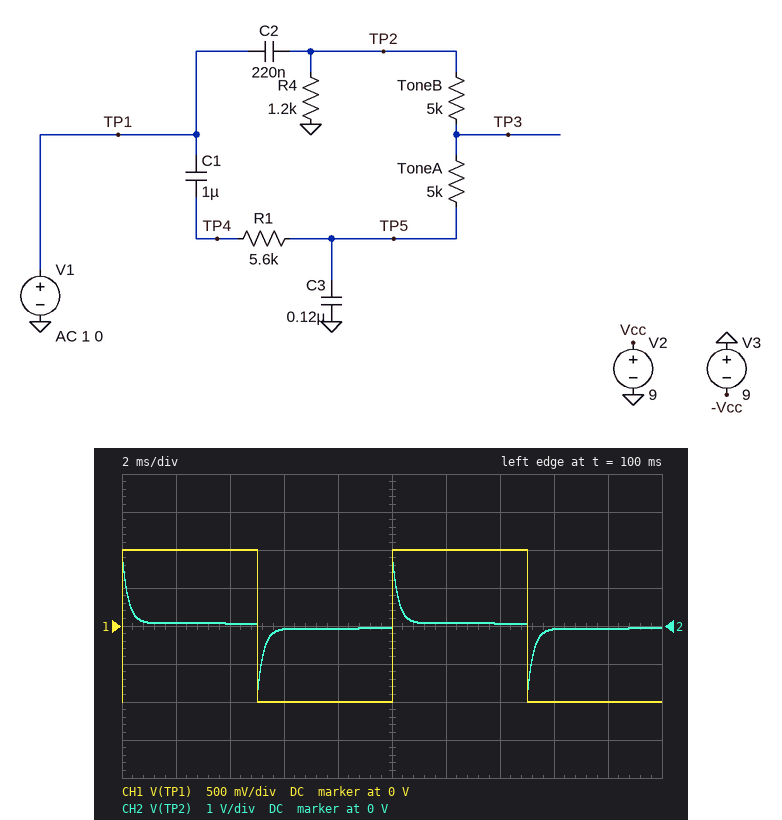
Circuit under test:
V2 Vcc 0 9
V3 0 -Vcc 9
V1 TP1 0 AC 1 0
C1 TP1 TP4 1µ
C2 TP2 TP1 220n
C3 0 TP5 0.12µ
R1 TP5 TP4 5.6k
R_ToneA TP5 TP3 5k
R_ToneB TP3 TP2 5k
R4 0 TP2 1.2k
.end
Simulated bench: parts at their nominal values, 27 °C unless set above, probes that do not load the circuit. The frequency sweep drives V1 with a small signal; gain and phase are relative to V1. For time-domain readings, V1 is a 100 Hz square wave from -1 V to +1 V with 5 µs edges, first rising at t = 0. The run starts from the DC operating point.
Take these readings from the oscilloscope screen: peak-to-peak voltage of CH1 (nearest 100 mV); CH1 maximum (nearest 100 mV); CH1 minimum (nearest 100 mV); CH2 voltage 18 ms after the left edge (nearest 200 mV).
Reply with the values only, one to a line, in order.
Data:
2.0 V
1.0 V
-1.0 V
0 V
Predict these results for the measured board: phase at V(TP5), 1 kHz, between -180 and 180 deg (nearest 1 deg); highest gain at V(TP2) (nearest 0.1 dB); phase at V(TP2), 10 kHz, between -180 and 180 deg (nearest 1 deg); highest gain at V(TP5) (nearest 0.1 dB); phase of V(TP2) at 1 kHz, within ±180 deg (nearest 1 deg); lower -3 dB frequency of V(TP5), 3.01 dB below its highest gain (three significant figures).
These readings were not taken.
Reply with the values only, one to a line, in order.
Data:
-58 deg
0 dB
4 deg
-4.0 dB
33 deg
8.64 Hz
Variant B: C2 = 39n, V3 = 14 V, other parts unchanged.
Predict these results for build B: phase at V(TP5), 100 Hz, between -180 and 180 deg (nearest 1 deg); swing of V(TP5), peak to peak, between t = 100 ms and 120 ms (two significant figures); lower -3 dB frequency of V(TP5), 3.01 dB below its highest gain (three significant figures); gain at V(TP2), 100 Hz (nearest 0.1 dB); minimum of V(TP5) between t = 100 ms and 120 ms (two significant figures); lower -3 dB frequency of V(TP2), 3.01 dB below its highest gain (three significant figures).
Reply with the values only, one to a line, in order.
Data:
-9 deg
1.3 V
8.58 Hz
-23.5 dB
-650 mV
3.87 kHz
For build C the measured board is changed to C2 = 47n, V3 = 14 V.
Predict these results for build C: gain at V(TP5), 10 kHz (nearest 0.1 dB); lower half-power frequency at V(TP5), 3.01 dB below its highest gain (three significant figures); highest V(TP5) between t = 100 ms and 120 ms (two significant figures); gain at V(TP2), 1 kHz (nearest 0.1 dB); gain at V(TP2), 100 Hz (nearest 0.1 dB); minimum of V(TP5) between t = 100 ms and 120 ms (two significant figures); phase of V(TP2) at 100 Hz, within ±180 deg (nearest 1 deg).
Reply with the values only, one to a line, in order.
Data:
-28.9 dB
8.58 Hz
650 mV
-11.0 dB
-23.3 dB
-650 mV
17 deg
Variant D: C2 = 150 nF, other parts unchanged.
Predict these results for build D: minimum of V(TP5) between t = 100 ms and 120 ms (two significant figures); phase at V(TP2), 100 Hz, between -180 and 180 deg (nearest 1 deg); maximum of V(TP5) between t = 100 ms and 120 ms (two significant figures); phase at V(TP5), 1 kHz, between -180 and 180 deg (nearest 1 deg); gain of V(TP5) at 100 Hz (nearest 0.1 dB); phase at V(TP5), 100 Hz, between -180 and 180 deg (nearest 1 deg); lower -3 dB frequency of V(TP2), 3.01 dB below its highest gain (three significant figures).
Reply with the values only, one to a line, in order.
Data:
-660 mV
49 deg
660 mV
-57 deg
-4.1 dB
-7 deg
1.04 kHz
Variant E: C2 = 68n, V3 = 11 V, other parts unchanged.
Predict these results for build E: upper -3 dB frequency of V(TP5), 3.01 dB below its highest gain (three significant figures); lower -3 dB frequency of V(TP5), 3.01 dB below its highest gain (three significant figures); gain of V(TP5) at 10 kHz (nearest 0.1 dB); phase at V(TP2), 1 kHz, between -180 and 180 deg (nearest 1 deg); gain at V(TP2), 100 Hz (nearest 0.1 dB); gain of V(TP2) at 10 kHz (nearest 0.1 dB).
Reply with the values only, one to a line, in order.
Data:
406 Hz
8.58 Hz
-28.8 dB
64 deg
-22.6 dB
-0.2 dB
